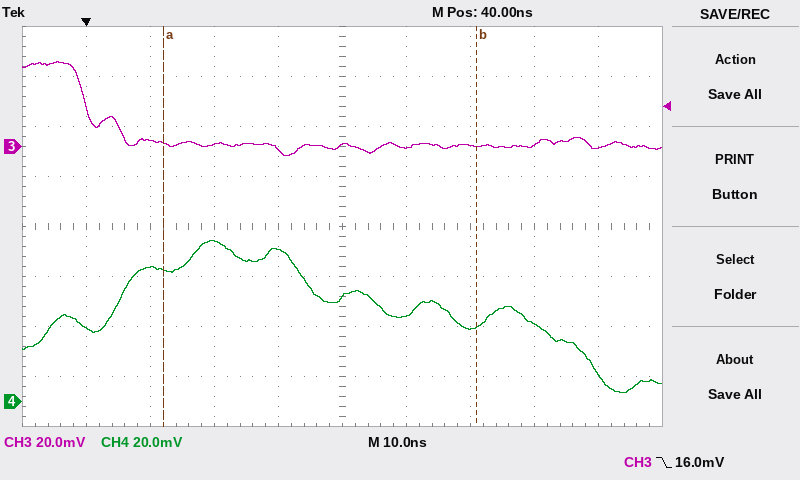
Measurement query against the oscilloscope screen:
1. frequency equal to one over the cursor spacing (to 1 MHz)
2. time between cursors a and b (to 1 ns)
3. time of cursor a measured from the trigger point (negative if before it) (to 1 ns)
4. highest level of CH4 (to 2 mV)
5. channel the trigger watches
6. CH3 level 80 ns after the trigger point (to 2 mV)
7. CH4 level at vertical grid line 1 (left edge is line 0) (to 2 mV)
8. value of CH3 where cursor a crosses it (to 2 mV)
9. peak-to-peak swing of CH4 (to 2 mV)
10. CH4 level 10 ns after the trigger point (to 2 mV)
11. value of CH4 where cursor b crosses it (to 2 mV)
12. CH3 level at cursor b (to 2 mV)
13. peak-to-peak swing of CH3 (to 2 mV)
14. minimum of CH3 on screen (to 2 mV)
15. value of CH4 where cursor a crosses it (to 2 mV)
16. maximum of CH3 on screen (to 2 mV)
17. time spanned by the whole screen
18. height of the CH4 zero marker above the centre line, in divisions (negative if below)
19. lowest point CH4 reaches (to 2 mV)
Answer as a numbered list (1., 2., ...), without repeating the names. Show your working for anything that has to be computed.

1. 1 / 49 ns ≈ 20 MHz
2. 49 ns
3. +12 ns
4. 64 mV
5. CH3
6. 0 mV
7. 30 mV
8. 2 mV
9. 64 mV − (4 mV) = 60 mV
10. 54 mV
11. 30 mV
12. 0 mV
13. 34 mV − (-4 mV) = 38 mV
14. -4 mV
15. 52 mV
16. 34 mV
17. 100 ns
18. -3.5 div
19. 4 mV
